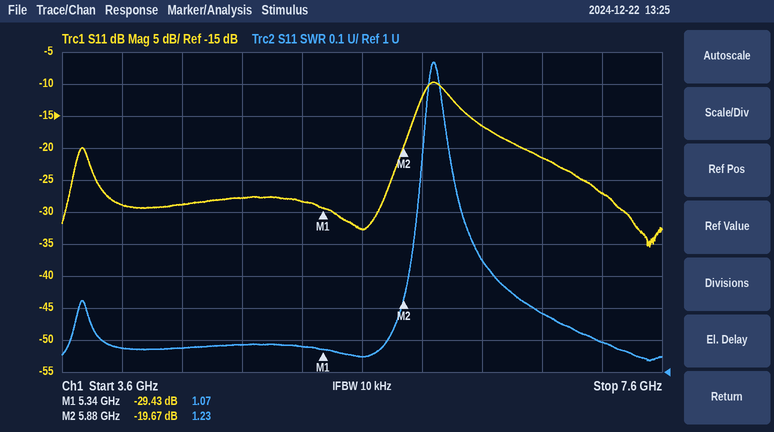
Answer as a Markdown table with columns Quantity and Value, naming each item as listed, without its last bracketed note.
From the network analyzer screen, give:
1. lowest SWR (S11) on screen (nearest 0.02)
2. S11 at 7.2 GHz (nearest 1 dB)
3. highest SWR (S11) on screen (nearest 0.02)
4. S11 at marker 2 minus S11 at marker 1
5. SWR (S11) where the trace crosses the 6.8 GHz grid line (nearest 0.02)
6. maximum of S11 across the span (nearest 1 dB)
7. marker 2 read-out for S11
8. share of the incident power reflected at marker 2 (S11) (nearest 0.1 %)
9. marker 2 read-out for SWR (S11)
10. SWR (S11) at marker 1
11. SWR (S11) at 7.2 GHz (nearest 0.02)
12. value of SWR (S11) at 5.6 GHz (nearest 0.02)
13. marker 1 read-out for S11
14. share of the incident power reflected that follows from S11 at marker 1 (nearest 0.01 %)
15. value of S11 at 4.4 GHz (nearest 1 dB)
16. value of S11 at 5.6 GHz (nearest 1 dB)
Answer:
| Quantity | Value |
|---|---|
| lowest SWR (S11) on screen | 1.04 |
| S11 at 7.2 GHz | -27 dB |
| highest SWR (S11) on screen | 1.96 |
| S11 at marker 2 minus S11 at marker 1 | 9.76 dB |
| SWR (S11) where the trace crosses the 6.8 GHz grid line | 1.18 |
| maximum of S11 across the span | -10 dB |
| marker 2 read-out for S11 | -19.67 dB |
| share of the incident power reflected at marker 2 (S11) | 1.1 % |
| marker 2 read-out for SWR | 1.23 |
| SWR (S11) at marker 1 | 1.07 |
| SWR (S11) at 7.2 GHz | 1.10 |
| value of SWR (S11) at 5.6 GHz | 1.04 |
| marker 1 read-out for S11 | -29.43 dB |
| share of the incident power reflected that follows from S11 at marker 1 | 0.11 % |
| value of S11 at 4.4 GHz | -29 dB |
| value of S11 at 5.6 GHz | -33 dB |
